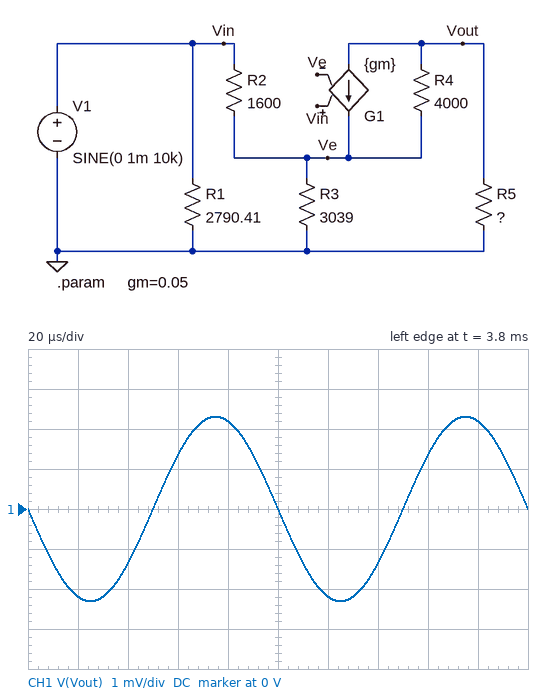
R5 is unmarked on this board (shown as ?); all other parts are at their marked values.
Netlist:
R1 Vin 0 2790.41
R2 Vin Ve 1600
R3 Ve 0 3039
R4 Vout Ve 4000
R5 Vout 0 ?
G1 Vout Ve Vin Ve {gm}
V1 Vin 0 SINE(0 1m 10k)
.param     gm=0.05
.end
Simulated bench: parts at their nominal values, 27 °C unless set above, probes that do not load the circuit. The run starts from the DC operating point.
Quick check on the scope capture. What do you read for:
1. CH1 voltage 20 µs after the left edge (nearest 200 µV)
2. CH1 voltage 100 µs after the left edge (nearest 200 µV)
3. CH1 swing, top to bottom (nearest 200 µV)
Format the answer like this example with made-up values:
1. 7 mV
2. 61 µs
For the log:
1. -2.2 mV
2. 0 V
3. 4.6 mV
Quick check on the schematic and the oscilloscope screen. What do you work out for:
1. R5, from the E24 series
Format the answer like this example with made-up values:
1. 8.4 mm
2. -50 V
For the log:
1. 7.5 kΩ
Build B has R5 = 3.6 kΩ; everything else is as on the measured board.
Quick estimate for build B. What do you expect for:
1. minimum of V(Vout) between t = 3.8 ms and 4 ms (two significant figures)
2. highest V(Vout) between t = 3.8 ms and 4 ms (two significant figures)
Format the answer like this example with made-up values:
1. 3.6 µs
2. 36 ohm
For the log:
1. -1.1 mV
2. 1.1 mV
